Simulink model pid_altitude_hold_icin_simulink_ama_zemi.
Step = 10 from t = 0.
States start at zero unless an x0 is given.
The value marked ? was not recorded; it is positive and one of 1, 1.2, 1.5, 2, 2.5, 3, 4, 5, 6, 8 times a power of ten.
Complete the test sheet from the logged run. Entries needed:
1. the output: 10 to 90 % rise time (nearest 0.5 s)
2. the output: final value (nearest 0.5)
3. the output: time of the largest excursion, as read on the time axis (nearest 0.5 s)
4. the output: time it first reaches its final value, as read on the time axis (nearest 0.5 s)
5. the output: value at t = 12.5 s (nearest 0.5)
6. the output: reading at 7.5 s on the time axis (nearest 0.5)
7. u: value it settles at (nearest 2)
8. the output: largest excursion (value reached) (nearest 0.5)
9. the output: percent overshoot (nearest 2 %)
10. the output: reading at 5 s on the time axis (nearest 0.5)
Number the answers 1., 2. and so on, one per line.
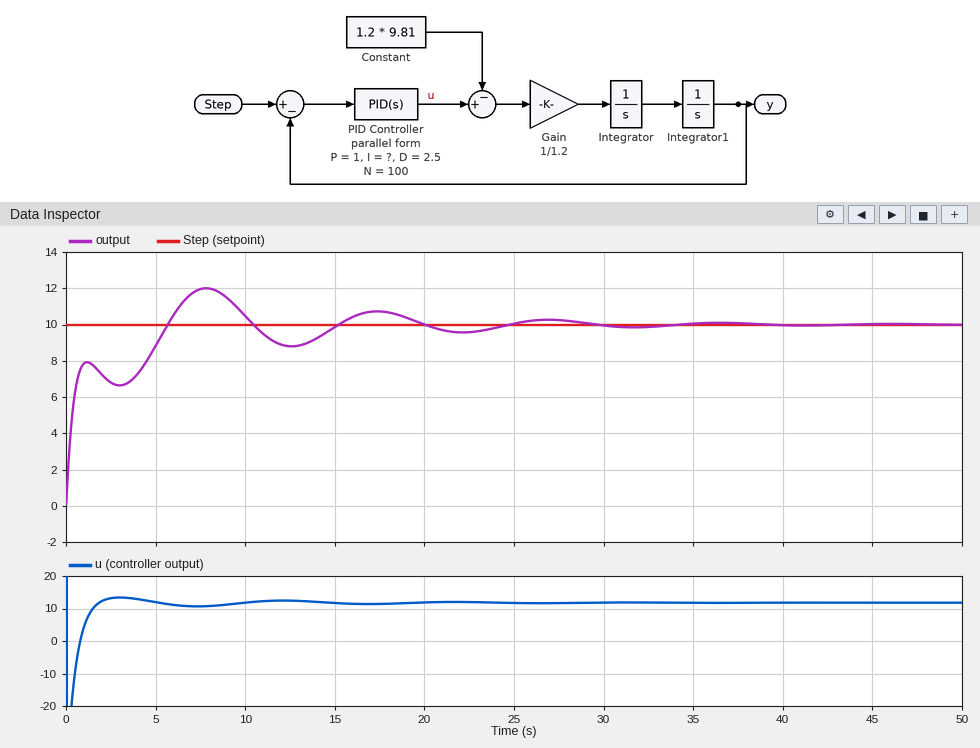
1. 5.0 s
2. 10.0
3. 8.0 s
4. 5.5 s
5. 9.0
6. 12.0
7. 12
8. 12.0
9. 20 %
10. 9.0
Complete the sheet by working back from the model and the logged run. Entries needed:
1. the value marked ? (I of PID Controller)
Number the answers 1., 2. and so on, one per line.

1. 1
